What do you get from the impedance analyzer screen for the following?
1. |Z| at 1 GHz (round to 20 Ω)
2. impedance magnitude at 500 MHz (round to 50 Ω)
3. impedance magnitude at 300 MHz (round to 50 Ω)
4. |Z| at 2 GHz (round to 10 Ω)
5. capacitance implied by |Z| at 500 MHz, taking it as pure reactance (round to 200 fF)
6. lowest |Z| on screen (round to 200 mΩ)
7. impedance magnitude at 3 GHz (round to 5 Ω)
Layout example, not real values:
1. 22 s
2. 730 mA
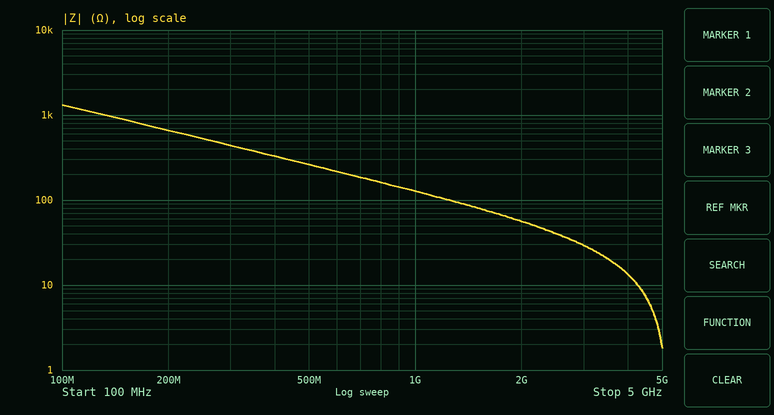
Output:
1. 120 Ω
2. 250 Ω
3. 450 Ω
4. 60 Ω
5. 1.2 pF
6. 1.8 Ω
7. 30 Ω
